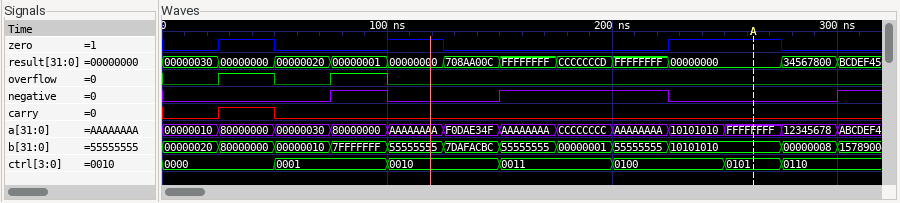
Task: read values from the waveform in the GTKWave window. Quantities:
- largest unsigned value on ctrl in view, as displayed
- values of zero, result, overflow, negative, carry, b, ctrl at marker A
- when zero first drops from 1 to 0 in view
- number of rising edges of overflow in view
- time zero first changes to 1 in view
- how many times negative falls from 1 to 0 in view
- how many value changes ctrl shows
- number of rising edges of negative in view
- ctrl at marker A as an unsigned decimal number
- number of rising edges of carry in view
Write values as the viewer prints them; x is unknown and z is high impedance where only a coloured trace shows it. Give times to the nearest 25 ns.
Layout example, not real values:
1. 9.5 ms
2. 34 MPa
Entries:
1. 0110
2. zero=1, result=00000000, overflow=0, negative=0, carry=0, b=10101010, ctrl=0101
3. 50 ns
4. 2
5. 25 ns
6. 2
7. 6
8. 3
9. 5
10. 1
